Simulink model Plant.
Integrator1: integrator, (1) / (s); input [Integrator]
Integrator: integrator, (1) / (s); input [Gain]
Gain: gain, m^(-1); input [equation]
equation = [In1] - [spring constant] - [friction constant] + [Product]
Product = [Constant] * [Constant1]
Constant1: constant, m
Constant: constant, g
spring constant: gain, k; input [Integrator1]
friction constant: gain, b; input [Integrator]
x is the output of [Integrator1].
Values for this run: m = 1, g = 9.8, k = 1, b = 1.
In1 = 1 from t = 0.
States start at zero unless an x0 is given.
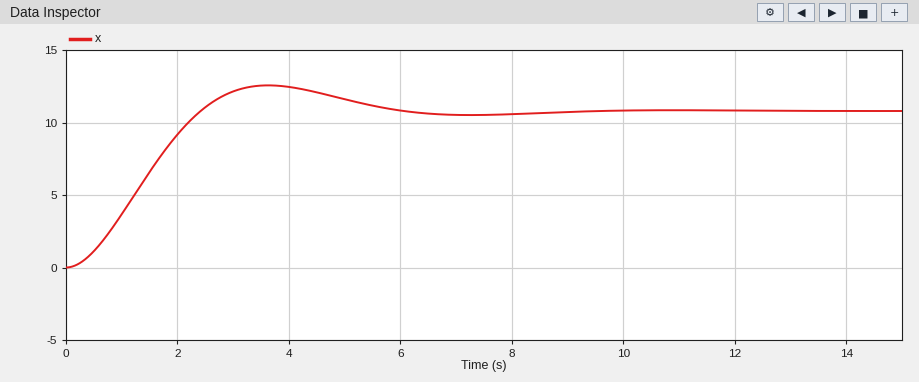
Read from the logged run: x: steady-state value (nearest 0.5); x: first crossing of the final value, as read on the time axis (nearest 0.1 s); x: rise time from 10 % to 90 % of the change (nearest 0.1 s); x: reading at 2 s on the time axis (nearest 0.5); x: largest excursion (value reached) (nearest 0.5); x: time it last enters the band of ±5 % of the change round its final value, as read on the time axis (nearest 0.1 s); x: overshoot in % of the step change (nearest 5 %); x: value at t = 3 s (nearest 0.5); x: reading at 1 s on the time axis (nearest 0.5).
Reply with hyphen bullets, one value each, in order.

- 11.0
- 2.4 s
- 1.6 s
- 9.0
- 12.5
- 5.3 s
- 15 %
- 12.0
- 3.5
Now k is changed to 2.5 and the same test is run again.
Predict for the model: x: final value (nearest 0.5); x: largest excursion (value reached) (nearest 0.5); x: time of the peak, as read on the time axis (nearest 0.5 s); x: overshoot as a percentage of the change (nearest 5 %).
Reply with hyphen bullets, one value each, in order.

- 4.5
- 6.0
- 2.0 s
- 35 %
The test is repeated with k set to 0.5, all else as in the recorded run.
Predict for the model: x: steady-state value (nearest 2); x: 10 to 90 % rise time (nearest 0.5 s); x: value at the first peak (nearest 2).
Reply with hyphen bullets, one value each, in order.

- 22
- 3.0 s
- 22
